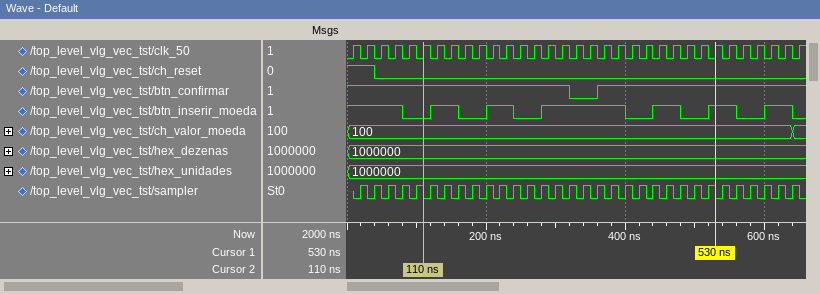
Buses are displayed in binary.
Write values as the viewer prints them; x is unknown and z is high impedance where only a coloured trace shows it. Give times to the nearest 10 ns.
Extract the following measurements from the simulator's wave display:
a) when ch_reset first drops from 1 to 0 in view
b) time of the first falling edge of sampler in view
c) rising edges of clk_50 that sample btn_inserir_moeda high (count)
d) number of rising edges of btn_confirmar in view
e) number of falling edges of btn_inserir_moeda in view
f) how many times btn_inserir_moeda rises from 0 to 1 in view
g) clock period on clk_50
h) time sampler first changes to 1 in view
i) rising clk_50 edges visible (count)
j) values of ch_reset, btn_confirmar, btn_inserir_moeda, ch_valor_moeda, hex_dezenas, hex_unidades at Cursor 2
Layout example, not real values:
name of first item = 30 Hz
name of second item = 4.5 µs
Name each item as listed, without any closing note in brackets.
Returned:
when ch_reset first drops from 1 to 0 in view = 40 ns
time of the first falling edge of sampler in view = 30 ns
rising edges of clk_50 that sample btn_inserir_moeda high = 20
number of rising edges of btn_confirmar in view = 1
number of falling edges of btn_inserir_moeda in view = 7
how many times btn_inserir_moeda rises from 0 to 1 in view = 6
clock period on clk_50 = 20 ns
time sampler first changes to 1 in view = 20 ns
rising clk_50 edges visible = 33
values of ch_reset, btn_confirmar, btn_inserir_moeda, ch_valor_moeda, hex_dezenas, hex_unidades at Cursor 2 = ch_reset=0, btn_confirmar=1, btn_inserir_moeda=0, ch_valor_moeda=100, hex_dezenas=1000000, hex_unidades=1000000
